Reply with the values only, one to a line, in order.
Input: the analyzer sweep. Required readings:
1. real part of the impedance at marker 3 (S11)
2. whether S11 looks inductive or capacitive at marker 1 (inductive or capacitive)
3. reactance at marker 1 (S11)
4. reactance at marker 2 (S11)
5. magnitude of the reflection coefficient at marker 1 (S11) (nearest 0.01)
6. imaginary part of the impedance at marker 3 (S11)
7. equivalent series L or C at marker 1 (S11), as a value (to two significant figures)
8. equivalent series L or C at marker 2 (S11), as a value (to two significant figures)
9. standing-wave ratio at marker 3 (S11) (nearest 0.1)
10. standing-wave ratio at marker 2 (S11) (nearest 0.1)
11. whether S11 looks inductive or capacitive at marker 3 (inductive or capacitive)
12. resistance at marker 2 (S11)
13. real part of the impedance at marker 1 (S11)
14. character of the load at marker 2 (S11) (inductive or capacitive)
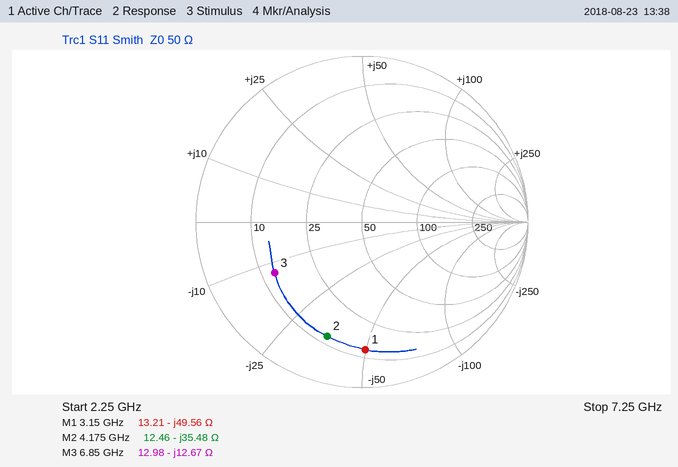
12.98 Ω
capacitive
-49.56 Ω
-35.48 Ω
0.77
-12.67 Ω
1.0 pF
1.1 pF
4.1
6.1
capacitive
12.46 Ω
13.21 Ω
capacitive
